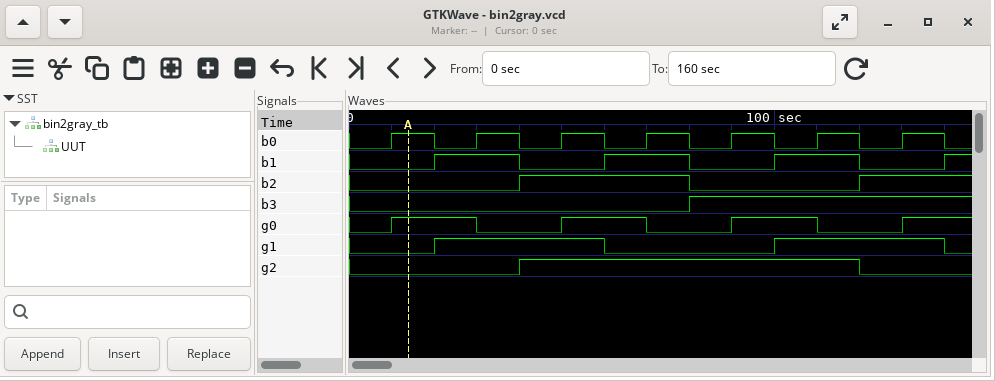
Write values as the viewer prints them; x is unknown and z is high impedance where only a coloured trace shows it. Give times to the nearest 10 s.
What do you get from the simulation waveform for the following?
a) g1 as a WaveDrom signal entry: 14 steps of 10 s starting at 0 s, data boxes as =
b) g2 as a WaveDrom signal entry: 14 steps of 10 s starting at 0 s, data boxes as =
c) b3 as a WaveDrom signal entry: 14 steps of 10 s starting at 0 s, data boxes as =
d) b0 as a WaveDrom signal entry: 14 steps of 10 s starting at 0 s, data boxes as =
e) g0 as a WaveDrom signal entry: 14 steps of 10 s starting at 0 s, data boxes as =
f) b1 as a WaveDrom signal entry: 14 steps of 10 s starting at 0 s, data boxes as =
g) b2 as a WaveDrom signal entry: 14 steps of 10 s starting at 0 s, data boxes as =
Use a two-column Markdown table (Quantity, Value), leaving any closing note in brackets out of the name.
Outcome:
| Quantity | Value |
|---|---|
| g1 as a WaveDrom signal entry: 14 steps of 10 s starting at 0 s, data boxes as = | {name: 'g1', wave: '0.1...0...1...'} |
| g2 as a WaveDrom signal entry: 14 steps of 10 s starting at 0 s, data boxes as = | {name: 'g2', wave: '0...1.......0.'} |
| b3 as a WaveDrom signal entry: 14 steps of 10 s starting at 0 s, data boxes as = | {name: 'b3', wave: '0.......1.....'} |
| b0 as a WaveDrom signal entry: 14 steps of 10 s starting at 0 s, data boxes as = | {name: 'b0', wave: '01010101010101'} |
| g0 as a WaveDrom signal entry: 14 steps of 10 s starting at 0 s, data boxes as = | {name: 'g0', wave: '01.0.1.0.1.0.1'} |
| b1 as a WaveDrom signal entry: 14 steps of 10 s starting at 0 s, data boxes as = | {name: 'b1', wave: '0.1.0.1.0.1.0.'} |
| b2 as a WaveDrom signal entry: 14 steps of 10 s starting at 0 s, data boxes as = | {name: 'b2', wave: '0...1...0...1.'} |
